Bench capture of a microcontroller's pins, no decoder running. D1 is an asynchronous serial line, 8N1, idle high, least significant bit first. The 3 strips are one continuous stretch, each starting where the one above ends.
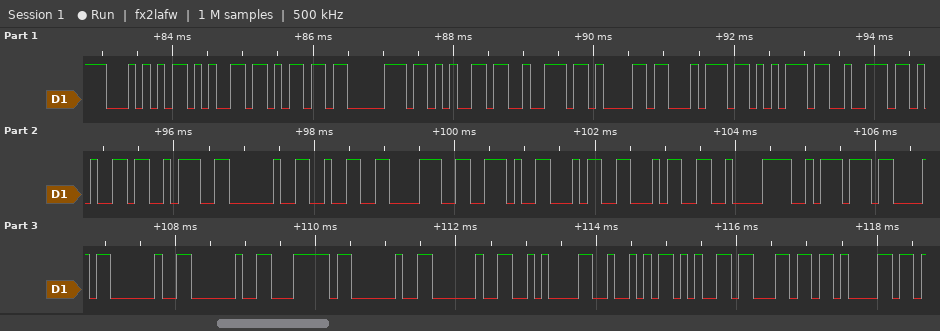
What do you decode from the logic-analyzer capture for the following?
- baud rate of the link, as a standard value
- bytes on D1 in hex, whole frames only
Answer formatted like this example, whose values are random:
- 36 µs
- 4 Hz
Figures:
- 9600 baud
- 54 65 6D 70 65 72 61 74 75 72 65 3A 20 32 38 2E 34 34 C2 BA 43 20 20 7C 20 20 0A 52 65 6C 61
